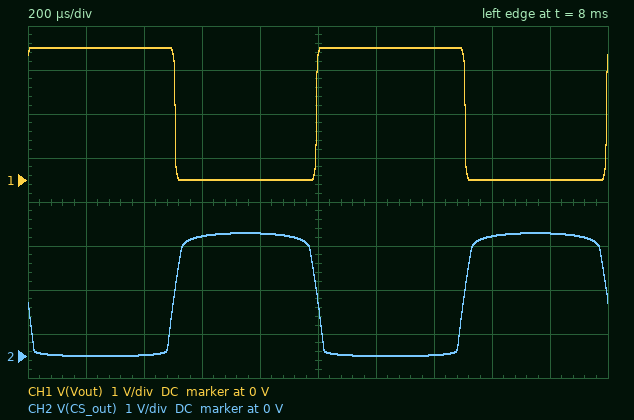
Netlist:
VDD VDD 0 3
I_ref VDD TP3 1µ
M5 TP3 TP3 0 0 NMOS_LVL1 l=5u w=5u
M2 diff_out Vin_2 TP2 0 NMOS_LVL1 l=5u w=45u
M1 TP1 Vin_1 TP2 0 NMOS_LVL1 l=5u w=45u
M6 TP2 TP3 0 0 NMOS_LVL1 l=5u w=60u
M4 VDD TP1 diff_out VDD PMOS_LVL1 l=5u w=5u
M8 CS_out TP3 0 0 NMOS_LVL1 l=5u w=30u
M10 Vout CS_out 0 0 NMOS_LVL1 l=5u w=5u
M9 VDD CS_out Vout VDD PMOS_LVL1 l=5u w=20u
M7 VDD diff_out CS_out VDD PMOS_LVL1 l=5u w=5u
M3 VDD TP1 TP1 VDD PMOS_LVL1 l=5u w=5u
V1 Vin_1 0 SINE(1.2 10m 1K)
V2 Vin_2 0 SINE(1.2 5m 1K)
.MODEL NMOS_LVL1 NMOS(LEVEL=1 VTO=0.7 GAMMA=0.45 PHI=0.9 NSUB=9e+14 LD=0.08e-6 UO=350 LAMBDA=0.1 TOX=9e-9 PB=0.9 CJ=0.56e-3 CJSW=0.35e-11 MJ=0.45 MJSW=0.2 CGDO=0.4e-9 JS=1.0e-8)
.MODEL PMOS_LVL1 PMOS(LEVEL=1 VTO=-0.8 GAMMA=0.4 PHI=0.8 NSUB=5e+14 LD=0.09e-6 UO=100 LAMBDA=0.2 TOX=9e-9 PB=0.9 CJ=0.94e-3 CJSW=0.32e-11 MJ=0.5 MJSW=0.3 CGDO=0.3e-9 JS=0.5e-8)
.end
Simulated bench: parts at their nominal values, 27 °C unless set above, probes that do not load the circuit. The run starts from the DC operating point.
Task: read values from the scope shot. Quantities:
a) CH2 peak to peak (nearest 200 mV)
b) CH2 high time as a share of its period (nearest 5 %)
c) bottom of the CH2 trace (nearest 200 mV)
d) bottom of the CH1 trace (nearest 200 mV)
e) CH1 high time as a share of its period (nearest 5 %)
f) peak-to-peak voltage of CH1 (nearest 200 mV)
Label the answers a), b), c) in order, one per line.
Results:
a) 2.8 V
b) 50 %
c) 0 V
d) 0 V
e) 50 %
f) 3.0 V
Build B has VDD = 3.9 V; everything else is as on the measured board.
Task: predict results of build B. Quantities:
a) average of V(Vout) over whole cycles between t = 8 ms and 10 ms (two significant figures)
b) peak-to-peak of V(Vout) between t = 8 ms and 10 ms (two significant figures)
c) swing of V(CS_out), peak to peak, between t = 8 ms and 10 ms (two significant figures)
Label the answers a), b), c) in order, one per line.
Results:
a) 2.0 V
b) 3.9 V
c) 3.7 V
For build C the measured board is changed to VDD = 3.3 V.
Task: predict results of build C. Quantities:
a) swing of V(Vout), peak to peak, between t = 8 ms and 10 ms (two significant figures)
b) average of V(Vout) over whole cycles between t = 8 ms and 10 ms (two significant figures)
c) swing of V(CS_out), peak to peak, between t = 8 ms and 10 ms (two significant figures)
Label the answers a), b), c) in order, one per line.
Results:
a) 3.3 V
b) 1.7 V
c) 3.1 V
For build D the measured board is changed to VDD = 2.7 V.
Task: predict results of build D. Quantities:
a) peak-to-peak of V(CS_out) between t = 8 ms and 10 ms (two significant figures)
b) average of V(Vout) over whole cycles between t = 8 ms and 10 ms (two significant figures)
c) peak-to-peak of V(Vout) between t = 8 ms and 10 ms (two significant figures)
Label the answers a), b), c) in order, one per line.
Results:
a) 2.5 V
b) 1.4 V
c) 2.7 V
